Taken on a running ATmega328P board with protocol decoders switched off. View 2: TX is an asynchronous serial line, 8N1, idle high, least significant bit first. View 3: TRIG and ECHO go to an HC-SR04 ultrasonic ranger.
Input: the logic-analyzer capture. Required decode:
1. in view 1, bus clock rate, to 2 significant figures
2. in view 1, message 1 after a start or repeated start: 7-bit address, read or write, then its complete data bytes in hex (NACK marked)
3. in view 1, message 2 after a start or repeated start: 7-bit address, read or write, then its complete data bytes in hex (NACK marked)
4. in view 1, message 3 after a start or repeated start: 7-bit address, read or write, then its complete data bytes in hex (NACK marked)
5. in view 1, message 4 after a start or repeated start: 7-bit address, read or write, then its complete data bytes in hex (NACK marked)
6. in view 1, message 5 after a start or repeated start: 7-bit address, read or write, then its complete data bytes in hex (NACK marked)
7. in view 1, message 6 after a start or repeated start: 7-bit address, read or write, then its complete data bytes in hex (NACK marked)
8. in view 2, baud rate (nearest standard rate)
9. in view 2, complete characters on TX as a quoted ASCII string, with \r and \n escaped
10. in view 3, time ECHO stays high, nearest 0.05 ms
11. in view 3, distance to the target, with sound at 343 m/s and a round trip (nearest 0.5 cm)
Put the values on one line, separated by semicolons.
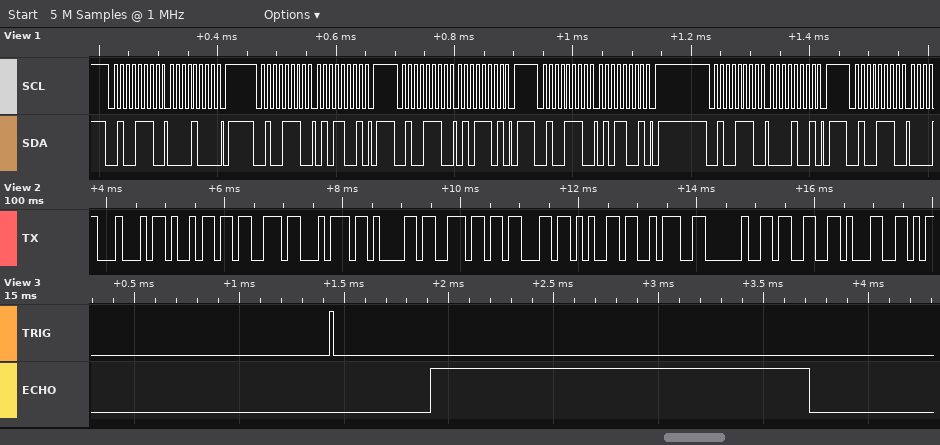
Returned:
100 kHz; 0x27 write: 08; 0x27 write: 59; 0x27 write: 5D; 0x27 write: 59; 0x27 write: 09; 0x27 write; 9600 baud; "Distance: 31"; 1.80 ms; 31 cm
